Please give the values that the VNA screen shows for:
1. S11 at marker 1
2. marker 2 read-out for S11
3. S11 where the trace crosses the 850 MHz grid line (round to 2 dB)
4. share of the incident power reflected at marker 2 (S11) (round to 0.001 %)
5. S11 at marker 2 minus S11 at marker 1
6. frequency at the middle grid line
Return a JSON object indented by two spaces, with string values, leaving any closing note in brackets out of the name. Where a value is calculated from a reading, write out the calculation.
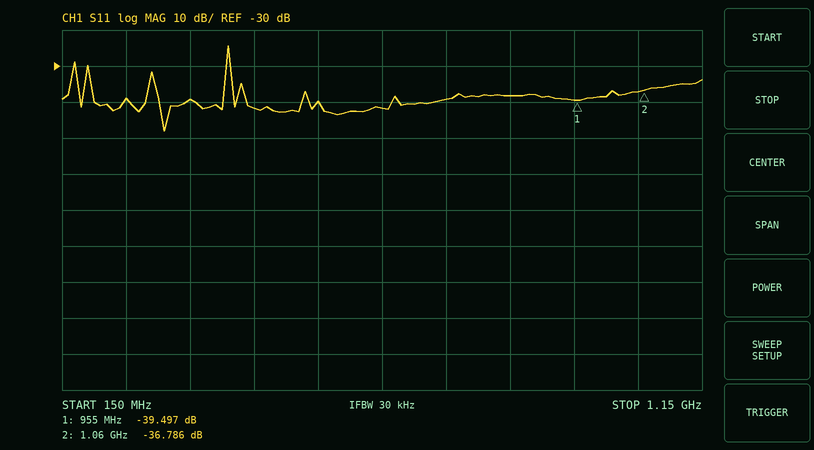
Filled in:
{
  "S11 at marker 1": "-39.497 dB",
  "marker 2 read-out for S11": "-36.786 dB",
  "S11 where the trace crosses the 850 MHz grid line": "-38 dB",
  "share of the incident power reflected at marker 2 (S11)": "10^(-36.786/10) ≈ 0.021 %",
  "S11 at marker 2 minus S11 at marker 1": "-36.786 − (-39.497) = 2.711 dB",
  "frequency at the middle grid line": "650 MHz"
}
